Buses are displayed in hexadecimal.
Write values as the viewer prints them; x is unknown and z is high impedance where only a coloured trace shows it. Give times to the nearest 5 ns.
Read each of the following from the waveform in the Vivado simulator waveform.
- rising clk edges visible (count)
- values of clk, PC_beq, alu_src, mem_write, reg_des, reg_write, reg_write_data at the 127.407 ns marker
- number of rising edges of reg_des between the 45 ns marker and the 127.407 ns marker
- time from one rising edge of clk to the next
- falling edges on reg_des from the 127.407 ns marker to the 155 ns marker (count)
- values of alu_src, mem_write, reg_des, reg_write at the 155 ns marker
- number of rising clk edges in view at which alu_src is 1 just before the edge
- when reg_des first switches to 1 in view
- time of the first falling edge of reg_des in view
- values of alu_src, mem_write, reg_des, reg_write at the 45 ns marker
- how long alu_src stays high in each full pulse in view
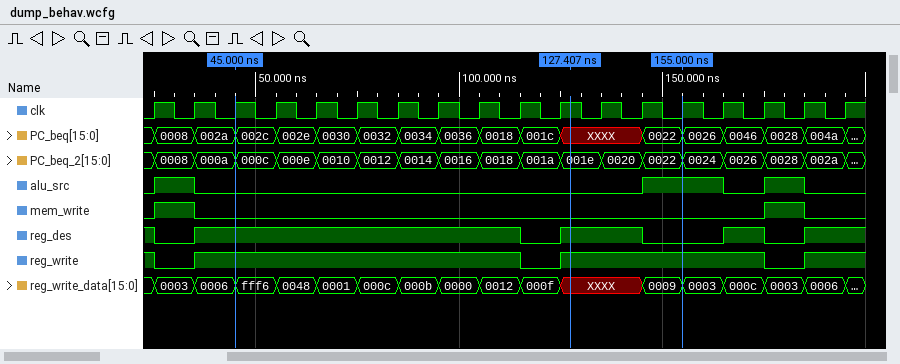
18
clk=1, PC_beq=XXXX, alu_src=0, mem_write=0, reg_des=1, reg_write=1, reg_write_data=XXXX
1
10 ns
1
alu_src=1, mem_write=0, reg_des=0, reg_write=1
4
35 ns
25 ns
alu_src=0, mem_write=0, reg_des=1, reg_write=1
10 ns, 20 ns, 10 ns
